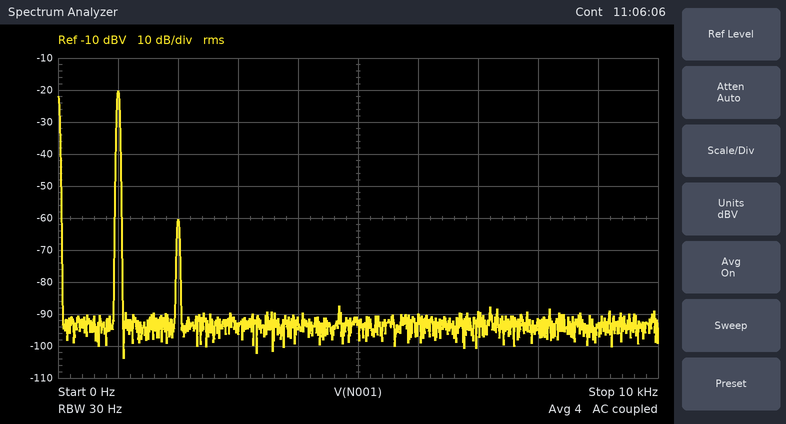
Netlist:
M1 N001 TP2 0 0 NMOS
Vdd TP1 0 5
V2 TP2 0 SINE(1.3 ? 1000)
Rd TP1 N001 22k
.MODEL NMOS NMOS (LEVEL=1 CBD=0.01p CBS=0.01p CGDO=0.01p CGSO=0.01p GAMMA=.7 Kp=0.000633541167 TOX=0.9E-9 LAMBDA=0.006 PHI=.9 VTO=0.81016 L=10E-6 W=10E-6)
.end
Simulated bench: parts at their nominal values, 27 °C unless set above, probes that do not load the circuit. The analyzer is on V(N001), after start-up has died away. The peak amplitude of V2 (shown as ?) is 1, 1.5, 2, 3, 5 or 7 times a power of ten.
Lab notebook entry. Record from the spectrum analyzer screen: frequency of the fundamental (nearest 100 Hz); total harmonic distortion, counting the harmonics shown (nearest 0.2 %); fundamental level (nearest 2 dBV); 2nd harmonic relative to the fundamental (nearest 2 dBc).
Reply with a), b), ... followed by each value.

a) 1.0 kHz
b) 1.0 %
c) -20 dBV
d) -40 dBc
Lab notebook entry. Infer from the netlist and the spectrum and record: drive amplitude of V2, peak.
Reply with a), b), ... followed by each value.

a) 20 mV
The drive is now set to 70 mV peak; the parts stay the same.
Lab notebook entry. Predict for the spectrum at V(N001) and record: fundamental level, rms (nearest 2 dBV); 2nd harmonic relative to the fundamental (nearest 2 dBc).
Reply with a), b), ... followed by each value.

a) -10 dBV
b) -30 dBc
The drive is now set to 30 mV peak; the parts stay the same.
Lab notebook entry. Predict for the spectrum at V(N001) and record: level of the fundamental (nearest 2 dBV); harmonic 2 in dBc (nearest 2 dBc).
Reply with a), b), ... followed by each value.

a) -16 dBV
b) -36 dBc
